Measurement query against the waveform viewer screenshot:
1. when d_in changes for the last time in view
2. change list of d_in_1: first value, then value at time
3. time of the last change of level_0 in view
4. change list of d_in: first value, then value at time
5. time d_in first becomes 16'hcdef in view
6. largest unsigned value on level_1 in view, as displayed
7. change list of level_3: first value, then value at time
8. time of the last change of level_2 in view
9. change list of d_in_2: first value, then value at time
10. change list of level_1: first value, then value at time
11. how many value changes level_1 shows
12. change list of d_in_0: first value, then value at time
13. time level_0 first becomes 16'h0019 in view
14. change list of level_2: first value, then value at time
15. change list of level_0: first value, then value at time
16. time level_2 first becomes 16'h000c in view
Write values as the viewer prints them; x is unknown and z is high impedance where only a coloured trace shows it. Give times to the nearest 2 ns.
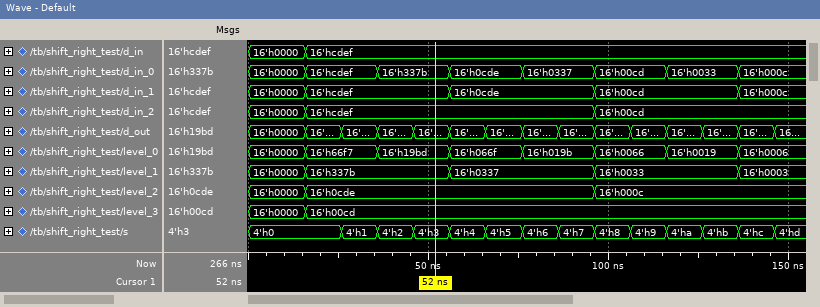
16 ns
16'h0000, 16'hcdef at 16 ns, 16'h0cde at 56 ns, 16'h00cd at 96 ns, 16'h000c at 136 ns
136 ns
16'h0000, 16'hcdef at 16 ns
16 ns
16'h337b
16'h0000, 16'h00cd at 16 ns
96 ns
16'h0000, 16'hcdef at 16 ns, 16'h00cd at 96 ns
16'h0000, 16'h337b at 16 ns, 16'h0337 at 56 ns, 16'h0033 at 96 ns, 16'h0003 at 136 ns
4
16'h0000, 16'hcdef at 16 ns, 16'h337b at 36 ns, 16'h0cde at 56 ns, 16'h0337 at 76 ns, 16'h00cd at 96 ns, 16'h0033 at 116 ns, 16'h000c at 136 ns
116 ns
16'h0000, 16'h0cde at 16 ns, 16'h000c at 96 ns
16'h0000, 16'h66f7 at 16 ns, 16'h19bd at 36 ns, 16'h066f at 56 ns, 16'h019b at 76 ns, 16'h0066 at 96 ns, 16'h0019 at 116 ns, 16'h0006 at 136 ns
96 ns
